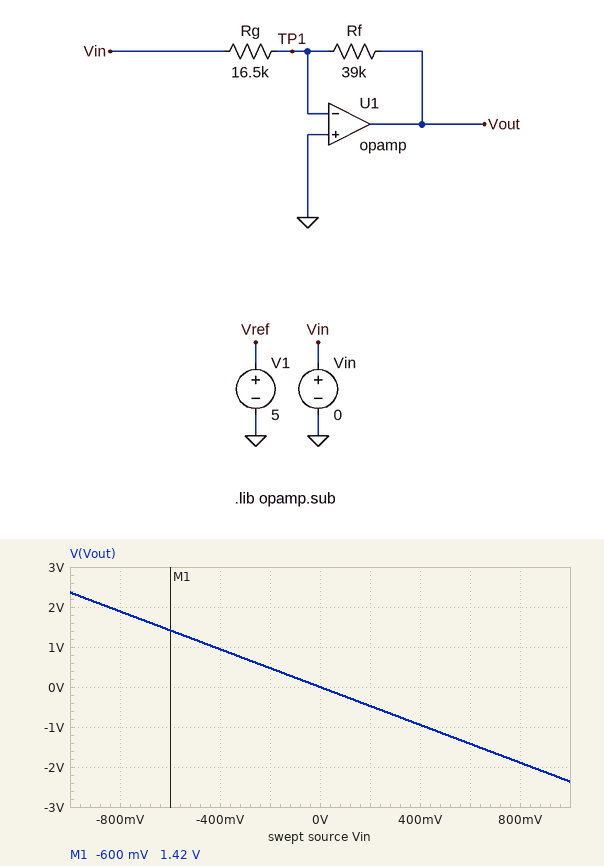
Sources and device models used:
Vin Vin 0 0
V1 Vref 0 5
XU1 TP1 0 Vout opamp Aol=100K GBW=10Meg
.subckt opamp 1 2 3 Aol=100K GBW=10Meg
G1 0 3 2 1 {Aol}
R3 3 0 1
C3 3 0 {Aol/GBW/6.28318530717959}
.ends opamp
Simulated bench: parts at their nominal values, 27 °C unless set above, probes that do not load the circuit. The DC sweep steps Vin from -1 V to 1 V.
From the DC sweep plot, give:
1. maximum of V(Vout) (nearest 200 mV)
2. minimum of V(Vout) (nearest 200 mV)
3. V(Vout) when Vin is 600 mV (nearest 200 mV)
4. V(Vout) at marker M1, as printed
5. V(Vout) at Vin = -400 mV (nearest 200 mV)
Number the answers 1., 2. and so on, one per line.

1. 2.4 V
2. -2.4 V
3. -1.4 V
4. 1.42 V
5. 1.0 V
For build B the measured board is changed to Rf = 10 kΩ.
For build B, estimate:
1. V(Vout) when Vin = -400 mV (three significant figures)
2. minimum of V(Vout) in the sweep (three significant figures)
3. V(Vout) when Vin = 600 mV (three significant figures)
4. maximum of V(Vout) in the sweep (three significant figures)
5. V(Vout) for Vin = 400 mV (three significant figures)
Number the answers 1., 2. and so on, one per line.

1. 242 mV
2. -606 mV
3. -364 mV
4. 606 mV
5. -242 mV
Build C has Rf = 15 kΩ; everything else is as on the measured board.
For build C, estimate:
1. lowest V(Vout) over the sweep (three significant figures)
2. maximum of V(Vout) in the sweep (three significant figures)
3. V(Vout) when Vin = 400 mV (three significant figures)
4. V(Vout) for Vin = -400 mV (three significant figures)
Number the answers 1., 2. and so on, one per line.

1. -909 mV
2. 909 mV
3. -364 mV
4. 364 mV
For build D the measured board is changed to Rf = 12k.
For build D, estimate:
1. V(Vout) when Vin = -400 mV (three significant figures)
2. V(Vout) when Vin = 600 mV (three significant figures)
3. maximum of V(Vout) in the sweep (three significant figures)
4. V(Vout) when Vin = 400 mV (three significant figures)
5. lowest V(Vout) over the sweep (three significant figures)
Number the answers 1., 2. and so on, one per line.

1. 291 mV
2. -436 mV
3. 727 mV
4. -291 mV
5. -727 mV
